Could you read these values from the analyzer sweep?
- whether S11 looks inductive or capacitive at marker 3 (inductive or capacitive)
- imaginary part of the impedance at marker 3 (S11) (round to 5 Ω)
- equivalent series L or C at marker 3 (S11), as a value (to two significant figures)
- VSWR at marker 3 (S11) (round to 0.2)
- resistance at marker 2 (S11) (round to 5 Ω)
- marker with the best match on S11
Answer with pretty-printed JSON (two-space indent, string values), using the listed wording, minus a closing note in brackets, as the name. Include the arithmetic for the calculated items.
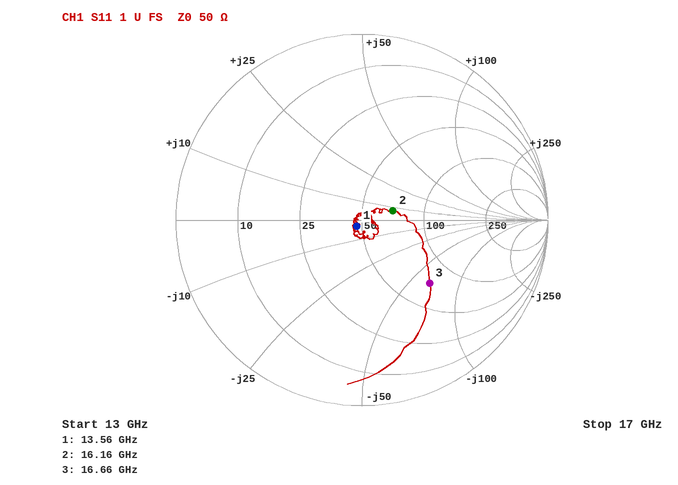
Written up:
{
  "whether S11 looks inductive or capacitive at marker 3": "capacitive",
  "imaginary part of the impedance at marker 3 (S11)": "-65 Ω",
  "equivalent series L or C at marker 3 (S11), as a value": "C = 1/(2π × 16.66 GHz × 65 Ω) ≈ 147 fF, so 150 fF to two significant figures",
  "VSWR at marker 3 (S11)": "3.0",
  "resistance at marker 2 (S11)": "70 Ω",
  "marker with the best match on S11": "marker 1"
}
